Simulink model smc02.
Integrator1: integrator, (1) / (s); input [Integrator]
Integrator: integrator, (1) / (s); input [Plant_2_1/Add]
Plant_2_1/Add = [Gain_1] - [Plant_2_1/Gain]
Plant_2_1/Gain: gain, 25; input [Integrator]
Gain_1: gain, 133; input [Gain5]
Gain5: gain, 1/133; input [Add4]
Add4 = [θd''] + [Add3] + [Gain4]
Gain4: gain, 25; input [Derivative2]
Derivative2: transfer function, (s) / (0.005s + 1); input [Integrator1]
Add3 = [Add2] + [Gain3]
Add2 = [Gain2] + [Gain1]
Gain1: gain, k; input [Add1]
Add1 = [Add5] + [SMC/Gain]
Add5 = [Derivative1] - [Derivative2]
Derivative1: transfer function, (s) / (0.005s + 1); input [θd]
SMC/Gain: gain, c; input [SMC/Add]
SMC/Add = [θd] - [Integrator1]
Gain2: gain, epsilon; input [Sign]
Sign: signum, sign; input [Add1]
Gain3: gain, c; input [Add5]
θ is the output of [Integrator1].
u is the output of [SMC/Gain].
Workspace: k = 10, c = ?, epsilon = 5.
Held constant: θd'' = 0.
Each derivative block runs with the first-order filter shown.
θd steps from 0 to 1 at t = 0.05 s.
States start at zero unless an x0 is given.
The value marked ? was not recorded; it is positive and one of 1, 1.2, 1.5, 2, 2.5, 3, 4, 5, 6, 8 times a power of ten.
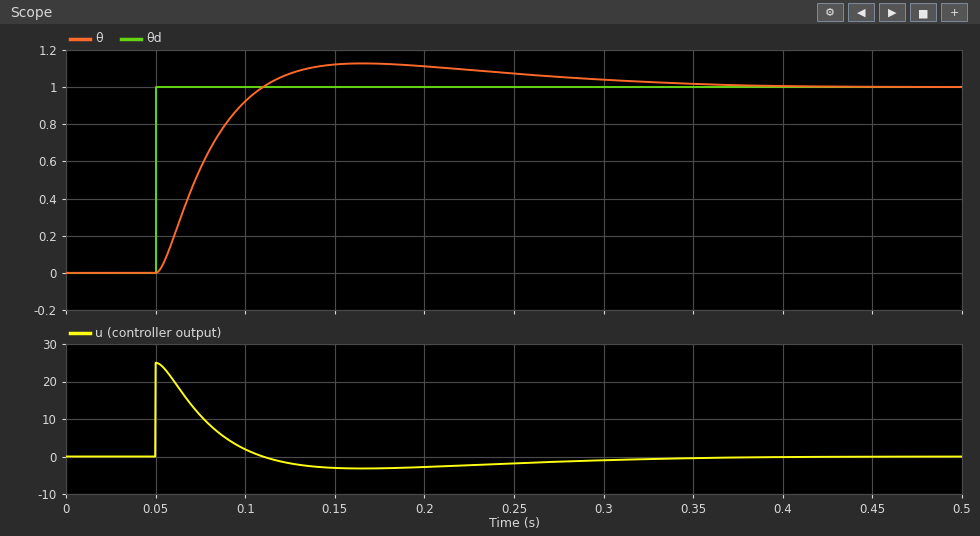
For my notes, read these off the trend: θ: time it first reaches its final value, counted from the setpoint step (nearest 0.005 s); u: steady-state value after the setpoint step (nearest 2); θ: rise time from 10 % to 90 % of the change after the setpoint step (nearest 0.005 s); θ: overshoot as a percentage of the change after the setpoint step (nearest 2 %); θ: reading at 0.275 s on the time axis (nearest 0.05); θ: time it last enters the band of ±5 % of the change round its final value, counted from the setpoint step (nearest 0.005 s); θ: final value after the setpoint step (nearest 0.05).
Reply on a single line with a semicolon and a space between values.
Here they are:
0.060 s; 0; 0.040 s; 12 %; 1.05; 0.235 s; 1.00
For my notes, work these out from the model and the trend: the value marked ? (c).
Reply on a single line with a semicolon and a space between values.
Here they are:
25
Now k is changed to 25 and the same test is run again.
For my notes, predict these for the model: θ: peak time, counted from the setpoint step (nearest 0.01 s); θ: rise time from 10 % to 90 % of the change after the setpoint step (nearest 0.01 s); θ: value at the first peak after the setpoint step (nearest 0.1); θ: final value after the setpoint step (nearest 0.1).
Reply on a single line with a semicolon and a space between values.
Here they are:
0.07 s; 0.03 s; 1.2; 1.0
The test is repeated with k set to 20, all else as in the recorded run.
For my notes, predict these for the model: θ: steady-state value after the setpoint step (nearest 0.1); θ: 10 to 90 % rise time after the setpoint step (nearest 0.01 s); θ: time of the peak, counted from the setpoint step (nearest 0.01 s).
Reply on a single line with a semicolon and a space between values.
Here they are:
1.0; 0.03 s; 0.08 s
